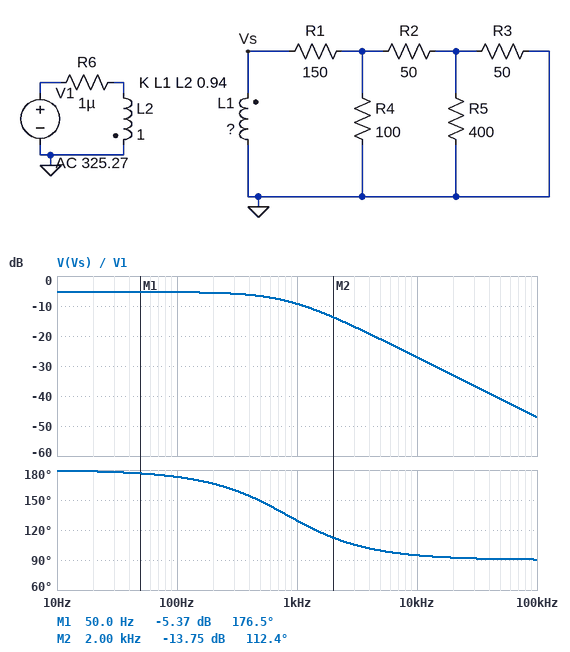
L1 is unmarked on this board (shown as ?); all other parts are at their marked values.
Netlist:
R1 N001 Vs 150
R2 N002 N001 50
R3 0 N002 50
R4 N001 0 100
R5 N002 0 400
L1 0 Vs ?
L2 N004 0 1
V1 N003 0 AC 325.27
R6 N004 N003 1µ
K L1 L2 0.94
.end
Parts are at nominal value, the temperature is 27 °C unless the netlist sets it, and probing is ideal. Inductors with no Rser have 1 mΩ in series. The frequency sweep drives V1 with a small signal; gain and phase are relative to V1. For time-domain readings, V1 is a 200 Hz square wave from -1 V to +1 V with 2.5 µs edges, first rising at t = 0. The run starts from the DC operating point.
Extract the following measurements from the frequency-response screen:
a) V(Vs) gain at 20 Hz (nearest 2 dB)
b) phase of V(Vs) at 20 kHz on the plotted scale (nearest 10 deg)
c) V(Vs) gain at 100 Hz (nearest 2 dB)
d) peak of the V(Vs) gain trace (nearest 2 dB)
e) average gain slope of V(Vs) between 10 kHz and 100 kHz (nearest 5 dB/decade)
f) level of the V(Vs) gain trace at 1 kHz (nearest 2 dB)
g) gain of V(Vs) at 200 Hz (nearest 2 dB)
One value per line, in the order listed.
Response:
-6 dB
90 deg
-6 dB
-6 dB
-20 dB/decade
-10 dB
-6 dB
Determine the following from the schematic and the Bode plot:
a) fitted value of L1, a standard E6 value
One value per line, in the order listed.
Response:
330 mH
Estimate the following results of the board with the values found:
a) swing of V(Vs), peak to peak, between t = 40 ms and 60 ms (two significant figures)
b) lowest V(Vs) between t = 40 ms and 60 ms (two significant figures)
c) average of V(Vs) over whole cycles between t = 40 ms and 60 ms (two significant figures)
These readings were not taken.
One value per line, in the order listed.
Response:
1.1 V
-1.1 V
-540 mV
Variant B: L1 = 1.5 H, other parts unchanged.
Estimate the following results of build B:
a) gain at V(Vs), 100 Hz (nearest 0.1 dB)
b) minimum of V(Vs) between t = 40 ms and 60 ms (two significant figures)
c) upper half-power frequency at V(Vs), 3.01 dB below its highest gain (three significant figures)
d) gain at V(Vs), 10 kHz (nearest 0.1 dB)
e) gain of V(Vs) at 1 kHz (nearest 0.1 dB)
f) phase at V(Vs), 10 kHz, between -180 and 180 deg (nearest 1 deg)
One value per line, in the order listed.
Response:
0.1 dB
-2.2 V
181 Hz
-33.6 dB
-13.8 dB
91 deg
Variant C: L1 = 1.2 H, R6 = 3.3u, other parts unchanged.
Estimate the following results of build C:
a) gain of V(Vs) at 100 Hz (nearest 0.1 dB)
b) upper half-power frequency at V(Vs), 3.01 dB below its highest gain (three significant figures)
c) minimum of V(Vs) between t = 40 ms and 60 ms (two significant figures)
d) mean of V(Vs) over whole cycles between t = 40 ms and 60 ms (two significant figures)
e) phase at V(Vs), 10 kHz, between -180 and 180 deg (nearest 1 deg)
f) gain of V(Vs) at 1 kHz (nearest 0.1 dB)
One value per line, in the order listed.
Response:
-0.5 dB
226 Hz
-2.0 V
-1.0 V
91 deg
-12.9 dB
